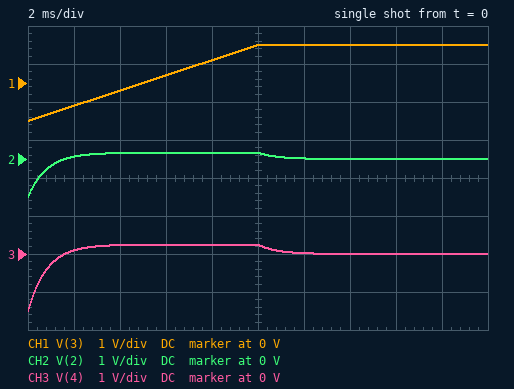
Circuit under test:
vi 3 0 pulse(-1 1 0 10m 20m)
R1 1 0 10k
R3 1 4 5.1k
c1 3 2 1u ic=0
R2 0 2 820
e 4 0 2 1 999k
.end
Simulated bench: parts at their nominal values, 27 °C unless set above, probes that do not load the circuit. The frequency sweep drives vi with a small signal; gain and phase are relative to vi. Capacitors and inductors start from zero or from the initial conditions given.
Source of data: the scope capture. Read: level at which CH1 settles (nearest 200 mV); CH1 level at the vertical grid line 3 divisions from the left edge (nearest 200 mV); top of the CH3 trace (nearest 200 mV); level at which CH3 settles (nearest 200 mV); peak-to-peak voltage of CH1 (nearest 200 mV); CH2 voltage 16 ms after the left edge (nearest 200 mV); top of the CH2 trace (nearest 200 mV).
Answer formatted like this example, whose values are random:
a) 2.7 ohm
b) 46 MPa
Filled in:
a) 1.0 V
b) 200 mV
c) 200 mV
d) 0 V
e) 2.0 V
f) 0 V
g) 200 mV
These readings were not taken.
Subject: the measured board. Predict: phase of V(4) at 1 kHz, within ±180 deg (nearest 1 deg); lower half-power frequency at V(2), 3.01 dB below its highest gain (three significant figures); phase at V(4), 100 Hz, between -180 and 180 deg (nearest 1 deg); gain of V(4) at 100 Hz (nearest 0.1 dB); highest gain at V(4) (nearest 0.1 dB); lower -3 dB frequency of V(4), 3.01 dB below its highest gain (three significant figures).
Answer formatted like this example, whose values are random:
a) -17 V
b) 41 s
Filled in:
a) 11 deg
b) 194 Hz
c) 63 deg
d) -3.2 dB
e) 3.6 dB
f) 194 Hz
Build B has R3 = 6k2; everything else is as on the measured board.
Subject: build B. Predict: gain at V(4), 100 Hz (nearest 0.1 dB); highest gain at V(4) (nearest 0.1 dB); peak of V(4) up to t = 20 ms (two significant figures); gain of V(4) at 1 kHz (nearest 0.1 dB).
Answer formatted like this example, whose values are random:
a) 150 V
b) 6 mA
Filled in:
a) -2.6 dB
b) 4.2 dB
c) 270 mV
d) 4.0 dB
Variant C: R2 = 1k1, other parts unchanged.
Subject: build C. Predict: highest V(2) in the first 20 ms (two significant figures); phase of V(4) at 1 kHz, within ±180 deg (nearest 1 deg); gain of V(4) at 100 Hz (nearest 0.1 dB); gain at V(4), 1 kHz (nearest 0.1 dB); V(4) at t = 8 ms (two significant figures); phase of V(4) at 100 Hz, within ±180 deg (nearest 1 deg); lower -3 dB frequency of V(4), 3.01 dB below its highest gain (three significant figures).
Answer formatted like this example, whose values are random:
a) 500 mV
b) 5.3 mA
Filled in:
a) 220 mV
b) 8 deg
c) -1.3 dB
d) 3.5 dB
e) 330 mV
f) 55 deg
g) 145 Hz
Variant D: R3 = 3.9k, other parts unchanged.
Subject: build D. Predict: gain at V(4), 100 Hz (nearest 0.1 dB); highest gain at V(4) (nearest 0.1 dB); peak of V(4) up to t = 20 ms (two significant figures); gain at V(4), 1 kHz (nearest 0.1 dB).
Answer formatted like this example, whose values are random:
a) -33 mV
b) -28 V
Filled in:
a) -3.9 dB
b) 2.9 dB
c) 230 mV
d) 2.7 dB
